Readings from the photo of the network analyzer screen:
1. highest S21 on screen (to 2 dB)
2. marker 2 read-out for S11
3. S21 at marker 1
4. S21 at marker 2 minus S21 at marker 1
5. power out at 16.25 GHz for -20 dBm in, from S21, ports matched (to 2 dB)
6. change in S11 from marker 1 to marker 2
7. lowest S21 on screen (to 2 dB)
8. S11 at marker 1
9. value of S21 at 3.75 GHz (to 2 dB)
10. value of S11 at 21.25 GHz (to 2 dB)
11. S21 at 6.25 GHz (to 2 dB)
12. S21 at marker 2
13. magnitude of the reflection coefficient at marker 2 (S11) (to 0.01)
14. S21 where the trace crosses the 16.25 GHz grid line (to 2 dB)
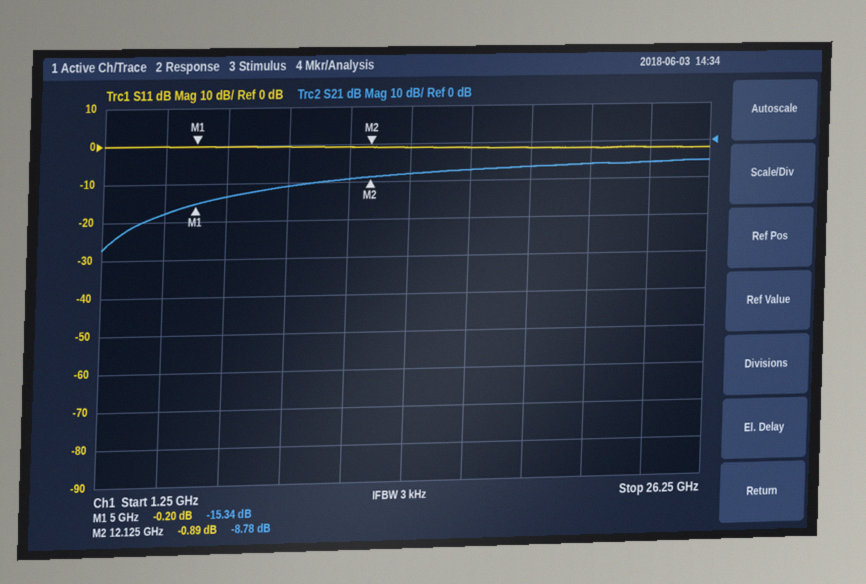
-6 dB
-0.89 dB
-15.34 dB
6.56 dB
-28 dBm
-0.69 dB
-28 dB
-0.20 dB
-18 dB
-2 dB
-14 dB
-8.78 dB
0.90
-8 dB
